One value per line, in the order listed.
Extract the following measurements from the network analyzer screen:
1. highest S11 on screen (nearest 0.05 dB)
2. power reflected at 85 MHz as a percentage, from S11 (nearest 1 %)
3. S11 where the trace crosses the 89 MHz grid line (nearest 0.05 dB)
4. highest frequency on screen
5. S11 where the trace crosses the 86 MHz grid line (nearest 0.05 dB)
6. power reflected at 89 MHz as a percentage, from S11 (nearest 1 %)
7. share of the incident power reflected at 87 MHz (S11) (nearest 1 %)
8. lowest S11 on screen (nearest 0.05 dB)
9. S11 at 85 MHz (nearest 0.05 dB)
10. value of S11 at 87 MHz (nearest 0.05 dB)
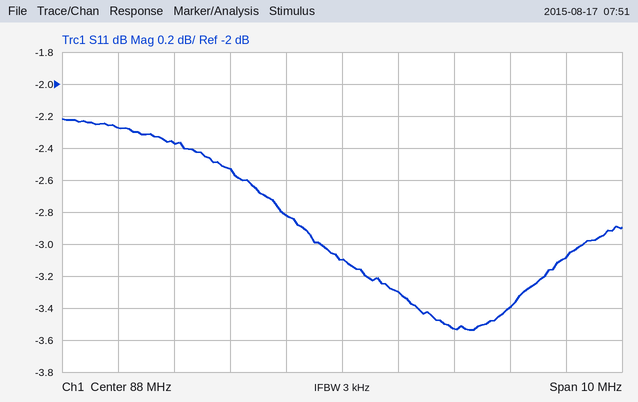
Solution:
-2.20 dB
58 %
-3.30 dB
93 MHz
-2.55 dB
47 %
52 %
-3.55 dB
-2.35 dB
-2.80 dB
